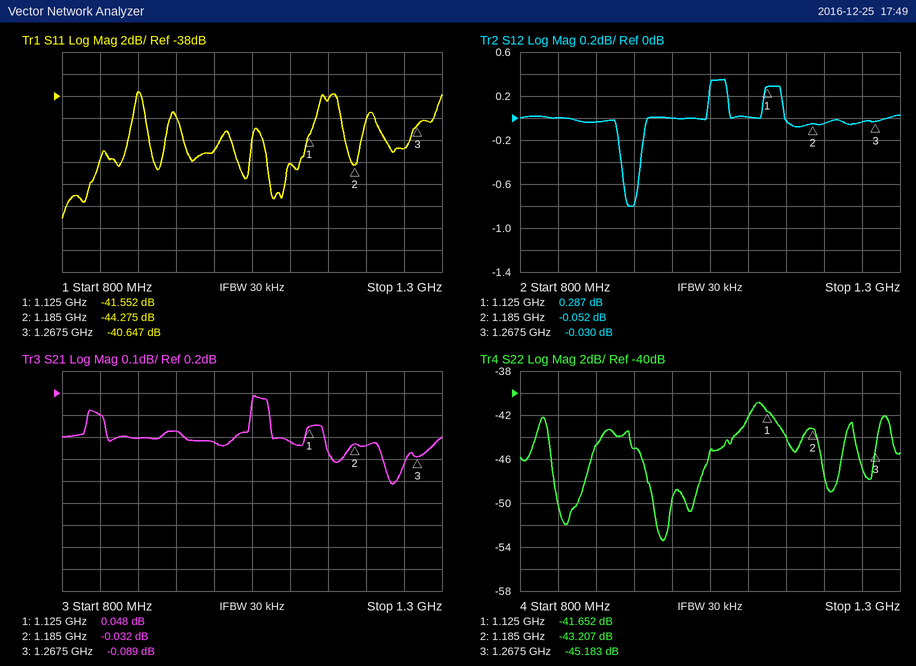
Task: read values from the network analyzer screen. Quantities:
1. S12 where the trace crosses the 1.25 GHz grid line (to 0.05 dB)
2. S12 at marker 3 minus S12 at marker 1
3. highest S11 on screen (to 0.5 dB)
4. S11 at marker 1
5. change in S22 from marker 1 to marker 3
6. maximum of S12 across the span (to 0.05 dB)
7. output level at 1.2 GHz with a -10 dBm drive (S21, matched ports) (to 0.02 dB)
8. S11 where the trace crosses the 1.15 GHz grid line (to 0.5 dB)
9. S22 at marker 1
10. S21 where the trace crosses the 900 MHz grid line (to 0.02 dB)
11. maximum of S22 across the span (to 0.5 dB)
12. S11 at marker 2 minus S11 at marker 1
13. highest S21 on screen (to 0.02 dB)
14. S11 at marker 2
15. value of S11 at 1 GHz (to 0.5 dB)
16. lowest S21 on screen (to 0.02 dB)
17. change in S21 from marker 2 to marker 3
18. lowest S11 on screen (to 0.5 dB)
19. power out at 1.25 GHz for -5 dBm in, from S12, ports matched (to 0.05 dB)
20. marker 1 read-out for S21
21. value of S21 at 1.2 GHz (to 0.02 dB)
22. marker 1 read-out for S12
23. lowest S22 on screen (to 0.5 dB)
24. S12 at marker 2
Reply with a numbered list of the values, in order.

1. -0.05 dB
2. -0.317 dB
3. -37.5 dB
4. -41.552 dB
5. -3.531 dB
6. 0.35 dB
7. -10.04 dBm
8. -38.5 dB
9. -41.652 dB
10. 0.00 dB
11. -41.0 dB
12. -2.723 dB
13. 0.18 dB
14. -44.275 dB
15. -43.0 dB
16. -0.22 dB
17. -0.057 dB
18. -49.0 dB
19. -5.05 dBm
20. 0.048 dB
21. -0.04 dB
22. 0.287 dB
23. -53.5 dB
24. -0.052 dB
